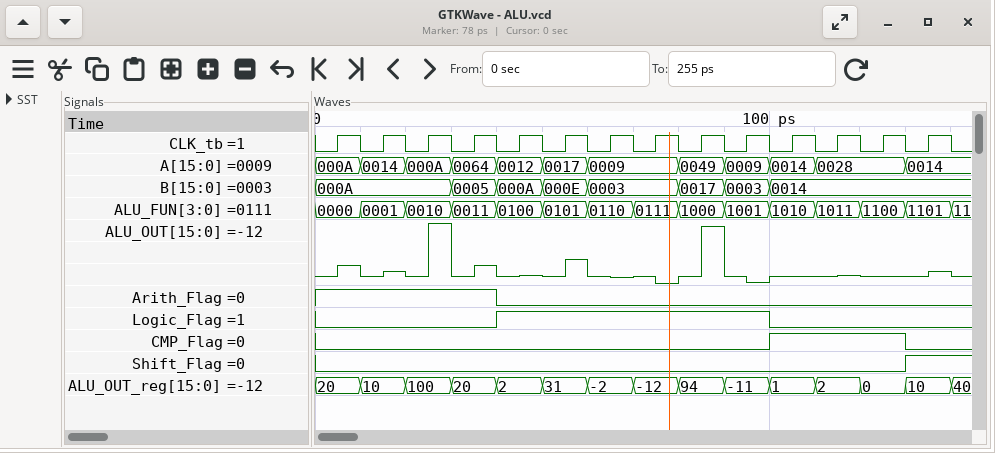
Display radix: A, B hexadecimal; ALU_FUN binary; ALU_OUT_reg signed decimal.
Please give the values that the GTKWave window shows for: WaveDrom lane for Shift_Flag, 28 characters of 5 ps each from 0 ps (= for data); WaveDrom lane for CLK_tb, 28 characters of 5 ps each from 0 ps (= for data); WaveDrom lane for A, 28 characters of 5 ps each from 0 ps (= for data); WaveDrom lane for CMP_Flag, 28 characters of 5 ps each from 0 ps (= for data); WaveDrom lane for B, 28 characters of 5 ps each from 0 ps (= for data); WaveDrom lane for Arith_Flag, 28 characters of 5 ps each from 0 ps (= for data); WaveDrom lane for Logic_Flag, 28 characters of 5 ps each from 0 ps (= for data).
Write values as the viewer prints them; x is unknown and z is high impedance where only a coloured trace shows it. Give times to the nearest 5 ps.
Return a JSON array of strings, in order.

["{name: 'Shift_Flag', wave: '0.........................1.'}", "{name: 'CLK_tb', wave: '0101010101010101010101010101'}", "{name: 'A', wave: '=.=.=.=.=.=.=...=.=.=.=...=.', data: '000A 0014 000A 0064 0012 0017 0009 0049 0009 0014 0028 0014'}", "{name: 'CMP_Flag', wave: '0...................1.....0.'}", "{name: 'B', wave: '=.....=.=.=.=...=.=.=.......', data: '000A 0005 000A 000E 0003 0017 0003 0014'}", "{name: 'Arith_Flag', wave: '1.......0...................'}", "{name: 'Logic_Flag', wave: '0.......1...........0.......'}"]
